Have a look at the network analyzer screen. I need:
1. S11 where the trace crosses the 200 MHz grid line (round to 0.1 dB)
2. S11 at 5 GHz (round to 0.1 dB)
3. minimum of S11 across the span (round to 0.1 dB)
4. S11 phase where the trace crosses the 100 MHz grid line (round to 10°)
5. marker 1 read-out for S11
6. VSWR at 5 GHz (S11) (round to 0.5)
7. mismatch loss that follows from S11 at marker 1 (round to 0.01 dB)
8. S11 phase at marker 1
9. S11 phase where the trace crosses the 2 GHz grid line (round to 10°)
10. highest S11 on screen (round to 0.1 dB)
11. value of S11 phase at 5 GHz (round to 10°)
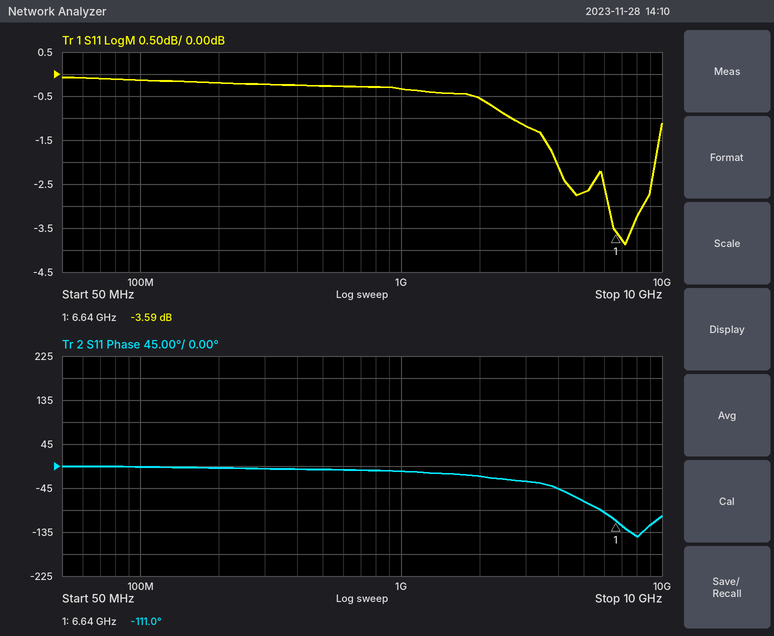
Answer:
-0.2 dB
-2.7 dB
-3.9 dB
0°
-3.59 dB
6.5
2.50 dB
-111.0°
-20°
-0.1 dB
-70°
